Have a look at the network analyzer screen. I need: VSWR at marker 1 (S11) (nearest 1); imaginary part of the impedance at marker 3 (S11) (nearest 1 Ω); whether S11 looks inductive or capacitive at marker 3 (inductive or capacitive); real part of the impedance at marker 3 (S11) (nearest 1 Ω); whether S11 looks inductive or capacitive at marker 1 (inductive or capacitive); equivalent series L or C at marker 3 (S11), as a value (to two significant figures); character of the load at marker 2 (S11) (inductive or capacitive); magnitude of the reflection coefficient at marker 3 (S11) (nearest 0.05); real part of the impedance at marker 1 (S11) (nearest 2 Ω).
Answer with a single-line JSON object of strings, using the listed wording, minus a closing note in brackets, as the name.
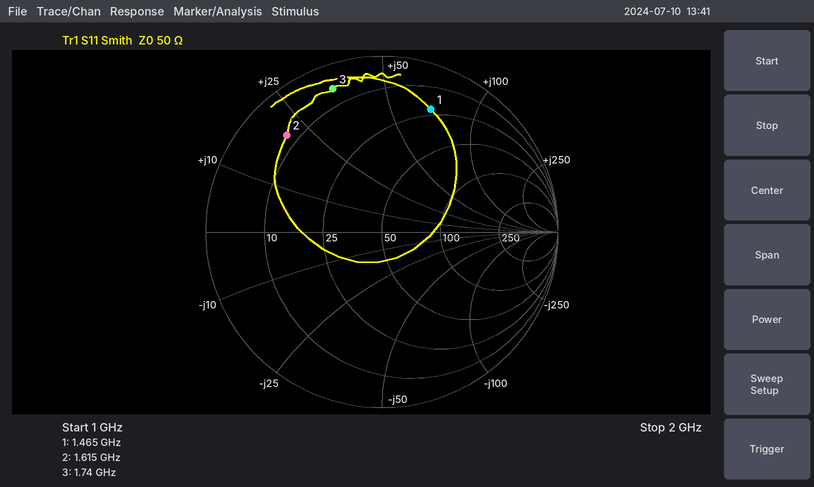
{"VSWR at marker 1 (S11)": "7", "imaginary part of the impedance at marker 3 (S11)": "+35 Ω", "whether S11 looks inductive or capacitive at marker 3": "inductive", "real part of the impedance at marker 3 (S11)": "6 Ω", "whether S11 looks inductive or capacitive at marker 1": "inductive", "equivalent series L or C at marker 3 (S11), as a value": "3.2 nH", "character of the load at marker 2 (S11)": "inductive", "magnitude of the reflection coefficient at marker 3 (S11)": "0.85", "real part of the impedance at marker 1 (S11)": "22 Ω"}
